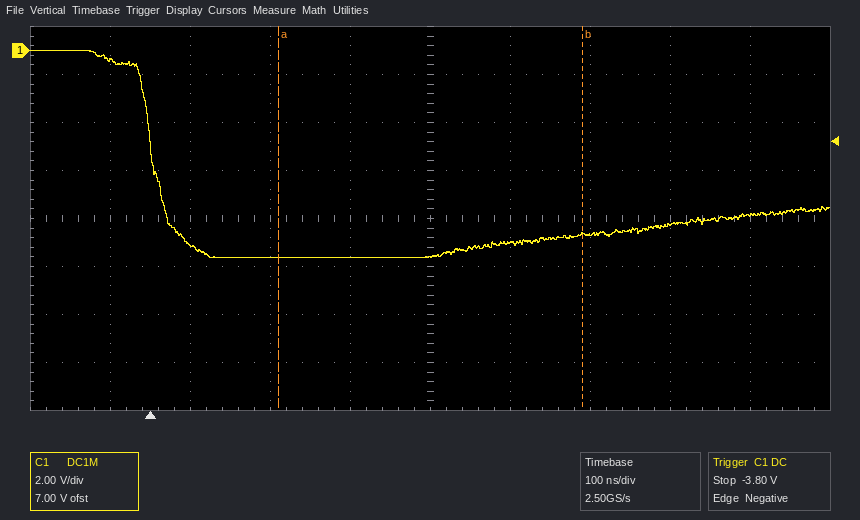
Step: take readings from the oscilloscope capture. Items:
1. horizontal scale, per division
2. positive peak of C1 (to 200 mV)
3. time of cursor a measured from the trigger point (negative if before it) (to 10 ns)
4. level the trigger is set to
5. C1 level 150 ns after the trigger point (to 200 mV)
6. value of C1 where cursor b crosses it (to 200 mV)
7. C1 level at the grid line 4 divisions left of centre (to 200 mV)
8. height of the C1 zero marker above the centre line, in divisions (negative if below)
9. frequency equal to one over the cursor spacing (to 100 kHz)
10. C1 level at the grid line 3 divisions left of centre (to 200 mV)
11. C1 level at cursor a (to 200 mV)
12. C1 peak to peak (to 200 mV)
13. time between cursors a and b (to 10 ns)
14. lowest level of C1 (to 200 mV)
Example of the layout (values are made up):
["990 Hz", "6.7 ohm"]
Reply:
["100 ns", "0.0 V", "+160 ns", "-3.80 V", "-8.6 V", "-7.6 V", "-400 mV", "+3.5 div", "2.6 MHz", "-8.0 V", "-8.6 V", "8.6 V", "380 ns", "-8.6 V"]
